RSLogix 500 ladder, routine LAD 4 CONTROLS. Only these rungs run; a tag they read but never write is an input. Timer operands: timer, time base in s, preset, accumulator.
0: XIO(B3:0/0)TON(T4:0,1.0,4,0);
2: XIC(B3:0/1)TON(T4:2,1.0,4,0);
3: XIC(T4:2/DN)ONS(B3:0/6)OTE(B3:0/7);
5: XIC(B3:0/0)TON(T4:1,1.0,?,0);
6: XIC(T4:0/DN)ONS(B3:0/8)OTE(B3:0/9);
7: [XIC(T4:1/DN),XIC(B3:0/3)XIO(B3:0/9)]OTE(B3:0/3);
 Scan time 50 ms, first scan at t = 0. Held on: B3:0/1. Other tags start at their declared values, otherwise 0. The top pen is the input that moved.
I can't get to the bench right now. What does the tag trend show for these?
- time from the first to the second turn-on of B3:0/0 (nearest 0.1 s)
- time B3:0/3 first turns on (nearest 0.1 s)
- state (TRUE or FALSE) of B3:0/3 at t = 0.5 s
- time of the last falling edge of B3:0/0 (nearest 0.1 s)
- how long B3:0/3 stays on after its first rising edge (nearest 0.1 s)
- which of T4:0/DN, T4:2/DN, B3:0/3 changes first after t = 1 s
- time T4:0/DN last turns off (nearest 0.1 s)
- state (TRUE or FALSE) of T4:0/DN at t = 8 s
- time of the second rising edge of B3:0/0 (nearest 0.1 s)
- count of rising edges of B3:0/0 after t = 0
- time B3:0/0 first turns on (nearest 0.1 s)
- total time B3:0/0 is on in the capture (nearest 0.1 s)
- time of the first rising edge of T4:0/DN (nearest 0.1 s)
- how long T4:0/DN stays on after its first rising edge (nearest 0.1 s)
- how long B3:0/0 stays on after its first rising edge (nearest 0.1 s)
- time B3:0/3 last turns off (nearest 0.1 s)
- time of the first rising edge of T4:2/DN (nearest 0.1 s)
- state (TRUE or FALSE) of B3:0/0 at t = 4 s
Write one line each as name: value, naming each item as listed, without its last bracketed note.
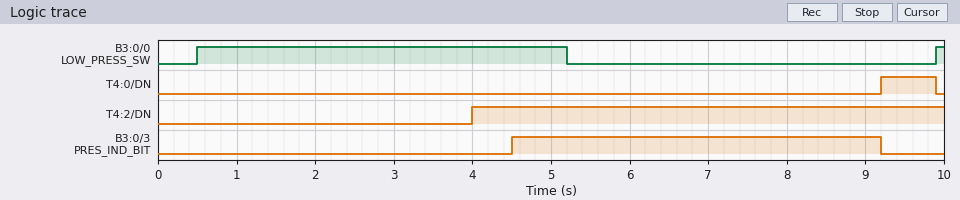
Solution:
time from the first to the second turn-on of B3:0/0: 9.4 s
time B3:0/3 first turns on: 4.5 s
state (TRUE or FALSE) of B3:0/3 at t = 0.5 s: FALSE
time of the last falling edge of B3:0/0: 5.2 s
how long B3:0/3 stays on after its first rising edge: 4.7 s
which of T4:0/DN, T4:2/DN, B3:0/3 changes first after t = 1 s: T4:2/DN
time T4:0/DN last turns off: 9.9 s
state (TRUE or FALSE) of T4:0/DN at t = 8 s: FALSE
time of the second rising edge of B3:0/0: 9.9 s
count of rising edges of B3:0/0 after t = 0: 2
time B3:0/0 first turns on: 0.5 s
total time B3:0/0 is on in the capture: 4.8 s
time of the first rising edge of T4:0/DN: 9.2 s
how long T4:0/DN stays on after its first rising edge: 0.7 s
how long B3:0/0 stays on after its first rising edge: 4.7 s
time B3:0/3 last turns off: 9.2 s
time of the first rising edge of T4:2/DN: 4.0 s
state (TRUE or FALSE) of B3:0/0 at t = 4 s: TRUE
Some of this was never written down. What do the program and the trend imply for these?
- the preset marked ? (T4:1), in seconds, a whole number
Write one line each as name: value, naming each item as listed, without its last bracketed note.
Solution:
the preset marked ? (T4:1), in seconds, a whole number: 4 s
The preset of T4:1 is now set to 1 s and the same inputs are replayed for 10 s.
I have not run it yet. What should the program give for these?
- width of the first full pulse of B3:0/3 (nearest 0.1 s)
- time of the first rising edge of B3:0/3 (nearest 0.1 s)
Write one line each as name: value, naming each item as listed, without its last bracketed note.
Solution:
width of the first full pulse of B3:0/3: 7.7 s
time of the first rising edge of B3:0/3: 1.5 s
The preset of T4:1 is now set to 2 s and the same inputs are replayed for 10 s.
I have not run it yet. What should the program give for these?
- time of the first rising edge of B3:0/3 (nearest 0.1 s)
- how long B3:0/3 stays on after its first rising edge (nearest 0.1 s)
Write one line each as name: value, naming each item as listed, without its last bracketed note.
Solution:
time of the first rising edge of B3:0/3: 2.5 s
how long B3:0/3 stays on after its first rising edge: 6.7 s
